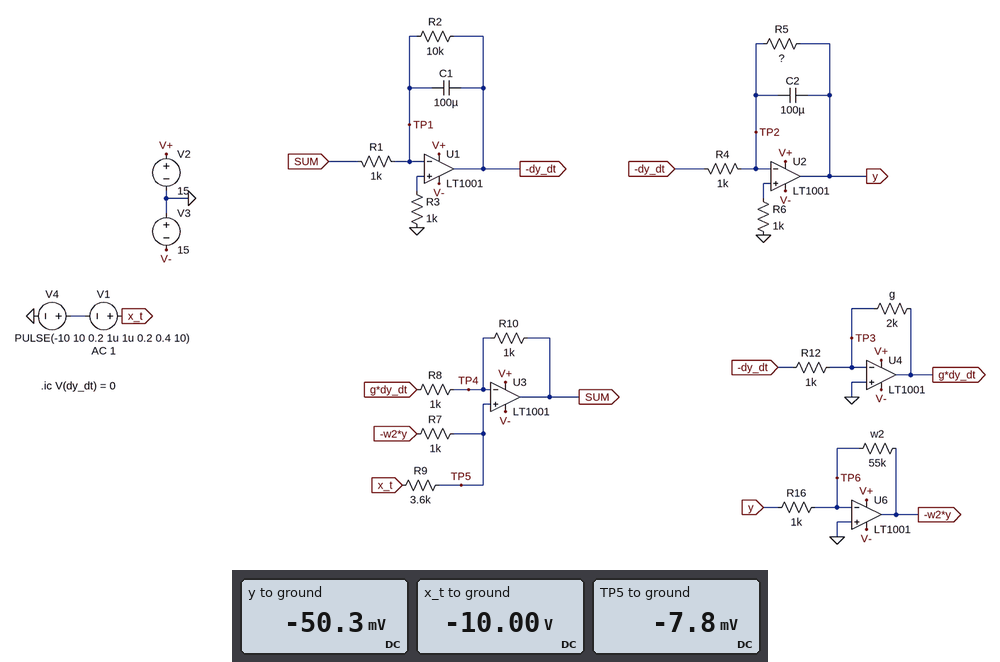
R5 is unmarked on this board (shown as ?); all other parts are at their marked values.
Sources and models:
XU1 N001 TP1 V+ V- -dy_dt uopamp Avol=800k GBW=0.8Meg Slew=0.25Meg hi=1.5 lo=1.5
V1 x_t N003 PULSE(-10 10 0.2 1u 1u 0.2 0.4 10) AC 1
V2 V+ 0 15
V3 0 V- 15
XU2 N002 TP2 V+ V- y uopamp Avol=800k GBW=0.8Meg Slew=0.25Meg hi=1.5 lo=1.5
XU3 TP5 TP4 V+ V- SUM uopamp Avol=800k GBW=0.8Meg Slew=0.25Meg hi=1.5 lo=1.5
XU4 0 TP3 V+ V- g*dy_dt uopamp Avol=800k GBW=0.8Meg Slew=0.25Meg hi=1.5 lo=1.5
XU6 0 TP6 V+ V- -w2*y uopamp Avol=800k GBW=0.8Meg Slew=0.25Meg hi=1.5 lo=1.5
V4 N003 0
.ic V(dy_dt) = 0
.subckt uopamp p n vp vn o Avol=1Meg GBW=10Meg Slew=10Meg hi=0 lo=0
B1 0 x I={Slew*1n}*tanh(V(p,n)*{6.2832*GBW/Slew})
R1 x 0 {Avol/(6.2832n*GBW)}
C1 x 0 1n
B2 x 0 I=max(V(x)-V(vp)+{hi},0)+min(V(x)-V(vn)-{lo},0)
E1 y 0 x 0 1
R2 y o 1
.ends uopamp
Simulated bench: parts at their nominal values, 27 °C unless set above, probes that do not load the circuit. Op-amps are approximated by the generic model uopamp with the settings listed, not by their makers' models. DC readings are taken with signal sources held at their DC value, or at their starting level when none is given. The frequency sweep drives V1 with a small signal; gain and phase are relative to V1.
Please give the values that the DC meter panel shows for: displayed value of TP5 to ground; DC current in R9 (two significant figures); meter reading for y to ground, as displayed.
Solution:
-7.8 mV
2.8 mA
-50.3 mV
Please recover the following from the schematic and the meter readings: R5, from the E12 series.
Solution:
6.8 kΩ
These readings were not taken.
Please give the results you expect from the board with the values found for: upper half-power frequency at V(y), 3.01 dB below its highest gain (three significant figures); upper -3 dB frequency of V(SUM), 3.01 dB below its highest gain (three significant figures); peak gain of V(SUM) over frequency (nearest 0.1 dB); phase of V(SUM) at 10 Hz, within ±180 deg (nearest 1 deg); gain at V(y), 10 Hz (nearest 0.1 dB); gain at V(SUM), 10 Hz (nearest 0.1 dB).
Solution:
16.3 Hz
17.3 Hz
5.2 dB
161 deg
-41.0 dB
-9.1 dB
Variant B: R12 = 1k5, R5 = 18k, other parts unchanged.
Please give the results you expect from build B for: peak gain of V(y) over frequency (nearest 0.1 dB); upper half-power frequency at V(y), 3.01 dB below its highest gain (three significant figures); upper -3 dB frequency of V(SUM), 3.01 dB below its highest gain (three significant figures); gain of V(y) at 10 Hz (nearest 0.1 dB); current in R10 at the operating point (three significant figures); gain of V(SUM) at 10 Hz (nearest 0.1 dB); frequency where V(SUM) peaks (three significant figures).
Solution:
-30.0 dB
15.8 Hz
16.2 Hz
-40.8 dB
1.73 µA
-8.9 dB
14.9 Hz
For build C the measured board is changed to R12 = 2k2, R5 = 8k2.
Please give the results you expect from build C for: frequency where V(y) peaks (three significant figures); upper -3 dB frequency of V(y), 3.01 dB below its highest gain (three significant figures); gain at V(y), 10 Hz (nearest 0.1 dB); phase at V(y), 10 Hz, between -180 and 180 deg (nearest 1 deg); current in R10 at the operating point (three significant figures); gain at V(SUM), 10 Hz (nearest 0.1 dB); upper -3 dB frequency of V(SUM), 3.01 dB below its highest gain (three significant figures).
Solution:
14.7 Hz
15.6 Hz
-40.7 dB
-9 deg
2.49 µA
-8.8 dB
15.8 Hz
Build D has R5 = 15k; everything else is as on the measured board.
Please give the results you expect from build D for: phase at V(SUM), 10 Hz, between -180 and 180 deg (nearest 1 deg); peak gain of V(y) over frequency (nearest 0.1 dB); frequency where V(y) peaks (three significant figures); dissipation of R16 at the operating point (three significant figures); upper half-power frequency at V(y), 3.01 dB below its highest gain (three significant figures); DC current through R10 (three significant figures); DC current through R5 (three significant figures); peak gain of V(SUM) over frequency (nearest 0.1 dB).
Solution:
162 deg
-33.2 dB
14.6 Hz
2.54 µW
16.2 Hz
3.19 µA
3.36 µA
5.5 dB
